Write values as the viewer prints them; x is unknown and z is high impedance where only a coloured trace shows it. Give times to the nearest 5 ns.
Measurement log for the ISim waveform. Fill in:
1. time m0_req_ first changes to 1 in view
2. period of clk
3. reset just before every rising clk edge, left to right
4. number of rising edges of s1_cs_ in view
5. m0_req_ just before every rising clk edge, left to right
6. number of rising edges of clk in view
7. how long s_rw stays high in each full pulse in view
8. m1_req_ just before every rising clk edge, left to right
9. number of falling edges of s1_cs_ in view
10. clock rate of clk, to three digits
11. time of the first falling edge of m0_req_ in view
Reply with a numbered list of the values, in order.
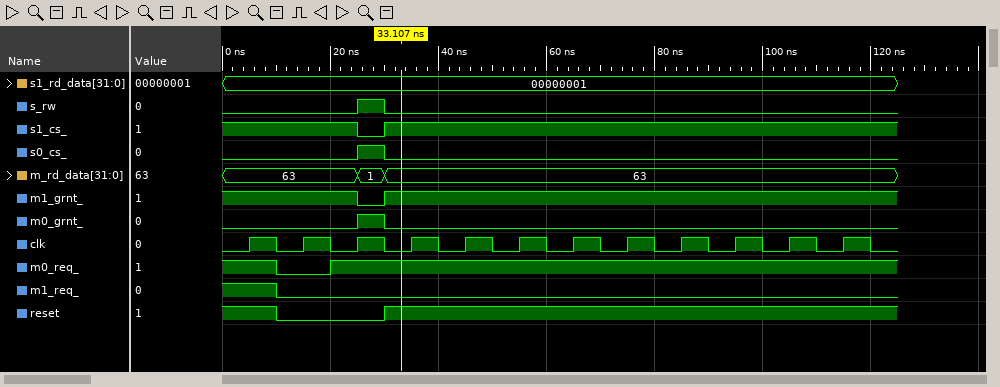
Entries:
1. 20 ns
2. 10 ns
3. 1 0 0 1 1 1 1 1 1 1 1 1
4. 1
5. 1 0 1 1 1 1 1 1 1 1 1 1
6. 12
7. 5 ns
8. 1 0 0 0 0 0 0 0 0 0 0 0
9. 1
10. 100 MHz
11. 10 ns
